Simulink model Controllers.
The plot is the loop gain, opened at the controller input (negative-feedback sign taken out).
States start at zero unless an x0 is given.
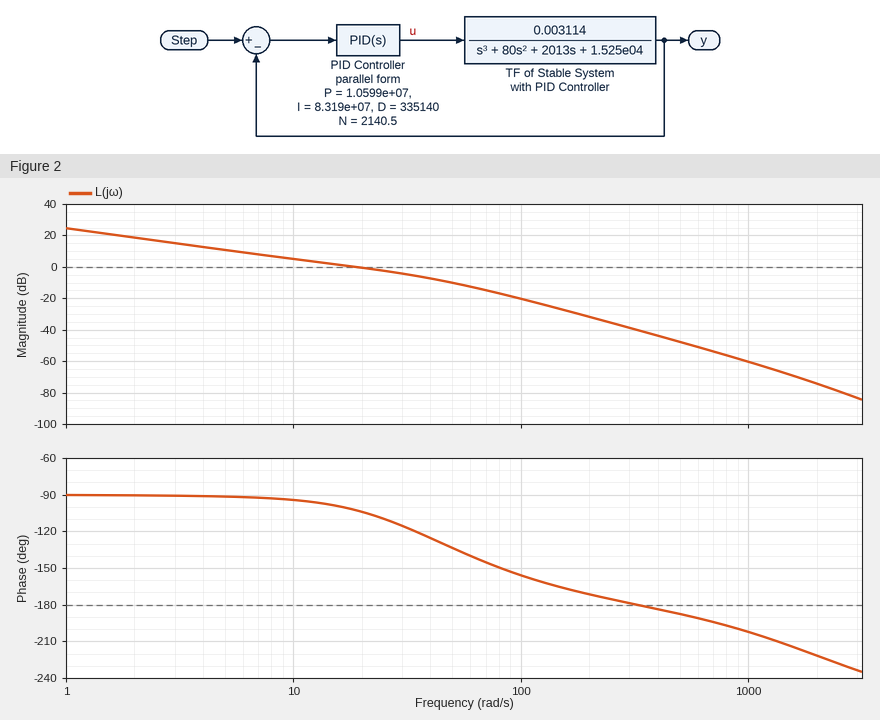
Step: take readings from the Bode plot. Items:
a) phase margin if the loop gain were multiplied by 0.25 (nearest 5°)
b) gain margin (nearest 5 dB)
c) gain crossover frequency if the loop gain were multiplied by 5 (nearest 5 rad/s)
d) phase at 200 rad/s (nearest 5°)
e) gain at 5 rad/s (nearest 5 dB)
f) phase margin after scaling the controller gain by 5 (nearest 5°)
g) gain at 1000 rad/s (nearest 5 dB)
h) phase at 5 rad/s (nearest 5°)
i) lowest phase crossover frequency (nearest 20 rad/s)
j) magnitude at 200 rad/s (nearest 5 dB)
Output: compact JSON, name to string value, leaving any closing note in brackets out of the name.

{"phase margin if the loop gain were multiplied by 0.25": "90°", "gain margin": "40 dB", "gain crossover frequency if the loop gain were multiplied by 5": "65 rad/s", "phase at 200 rad/s": "-170°", "gain at 5 rad/s": "10 dB", "phase margin after scaling the controller gain by 5": "35°", "gain at 1000 rad/s": "-60 dB", "phase at 5 rad/s": "-90°", "lowest phase crossover frequency": "320 rad/s", "magnitude at 200 rad/s": "-30 dB"}
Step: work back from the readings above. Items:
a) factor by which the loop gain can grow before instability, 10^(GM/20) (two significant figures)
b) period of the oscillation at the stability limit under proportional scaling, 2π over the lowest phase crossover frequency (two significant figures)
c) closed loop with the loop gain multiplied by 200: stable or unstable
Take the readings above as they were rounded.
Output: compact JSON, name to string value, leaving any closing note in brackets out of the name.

{"factor by which the loop gain can grow before instability, 10^(GM/20)": "100", "period of the oscillation at the stability limit under proportional scaling, 2π over the lowest phase crossover frequency": "0.020 s", "closed loop with the loop gain multiplied by 200: stable or unstable": "unstable"}
